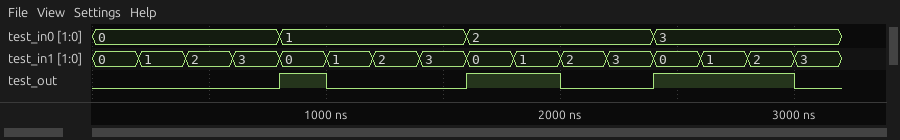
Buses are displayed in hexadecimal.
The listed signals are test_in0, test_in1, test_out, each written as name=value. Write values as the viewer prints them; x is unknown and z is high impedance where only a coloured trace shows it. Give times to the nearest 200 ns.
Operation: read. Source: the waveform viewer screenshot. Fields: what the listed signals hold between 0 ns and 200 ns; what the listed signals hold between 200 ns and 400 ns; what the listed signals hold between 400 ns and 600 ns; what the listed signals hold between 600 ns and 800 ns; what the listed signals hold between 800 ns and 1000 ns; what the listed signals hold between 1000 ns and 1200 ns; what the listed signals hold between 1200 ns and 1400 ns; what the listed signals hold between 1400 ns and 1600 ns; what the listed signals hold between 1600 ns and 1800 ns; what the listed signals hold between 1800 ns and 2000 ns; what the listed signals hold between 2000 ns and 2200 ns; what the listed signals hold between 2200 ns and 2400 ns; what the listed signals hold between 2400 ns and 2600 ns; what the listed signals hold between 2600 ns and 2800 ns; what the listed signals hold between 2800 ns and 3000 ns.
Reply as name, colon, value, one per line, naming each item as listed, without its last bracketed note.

what the listed signals hold between 0 ns and 200 ns: test_in0=0, test_in1=0, test_out=0
what the listed signals hold between 200 ns and 400 ns: test_in0=0, test_in1=1, test_out=0
what the listed signals hold between 400 ns and 600 ns: test_in0=0, test_in1=2, test_out=0
what the listed signals hold between 600 ns and 800 ns: test_in0=0, test_in1=3, test_out=0
what the listed signals hold between 800 ns and 1000 ns: test_in0=1, test_in1=0, test_out=1
what the listed signals hold between 1000 ns and 1200 ns: test_in0=1, test_in1=1, test_out=0
what the listed signals hold between 1200 ns and 1400 ns: test_in0=1, test_in1=2, test_out=0
what the listed signals hold between 1400 ns and 1600 ns: test_in0=1, test_in1=3, test_out=0
what the listed signals hold between 1600 ns and 1800 ns: test_in0=2, test_in1=0, test_out=1
what the listed signals hold between 1800 ns and 2000 ns: test_in0=2, test_in1=1, test_out=1
what the listed signals hold between 2000 ns and 2200 ns: test_in0=2, test_in1=2, test_out=0
what the listed signals hold between 2200 ns and 2400 ns: test_in0=2, test_in1=3, test_out=0
what the listed signals hold between 2400 ns and 2600 ns: test_in0=3, test_in1=0, test_out=1
what the listed signals hold between 2600 ns and 2800 ns: test_in0=3, test_in1=1, test_out=1
what the listed signals hold between 2800 ns and 3000 ns: test_in0=3, test_in1=2, test_out=1
